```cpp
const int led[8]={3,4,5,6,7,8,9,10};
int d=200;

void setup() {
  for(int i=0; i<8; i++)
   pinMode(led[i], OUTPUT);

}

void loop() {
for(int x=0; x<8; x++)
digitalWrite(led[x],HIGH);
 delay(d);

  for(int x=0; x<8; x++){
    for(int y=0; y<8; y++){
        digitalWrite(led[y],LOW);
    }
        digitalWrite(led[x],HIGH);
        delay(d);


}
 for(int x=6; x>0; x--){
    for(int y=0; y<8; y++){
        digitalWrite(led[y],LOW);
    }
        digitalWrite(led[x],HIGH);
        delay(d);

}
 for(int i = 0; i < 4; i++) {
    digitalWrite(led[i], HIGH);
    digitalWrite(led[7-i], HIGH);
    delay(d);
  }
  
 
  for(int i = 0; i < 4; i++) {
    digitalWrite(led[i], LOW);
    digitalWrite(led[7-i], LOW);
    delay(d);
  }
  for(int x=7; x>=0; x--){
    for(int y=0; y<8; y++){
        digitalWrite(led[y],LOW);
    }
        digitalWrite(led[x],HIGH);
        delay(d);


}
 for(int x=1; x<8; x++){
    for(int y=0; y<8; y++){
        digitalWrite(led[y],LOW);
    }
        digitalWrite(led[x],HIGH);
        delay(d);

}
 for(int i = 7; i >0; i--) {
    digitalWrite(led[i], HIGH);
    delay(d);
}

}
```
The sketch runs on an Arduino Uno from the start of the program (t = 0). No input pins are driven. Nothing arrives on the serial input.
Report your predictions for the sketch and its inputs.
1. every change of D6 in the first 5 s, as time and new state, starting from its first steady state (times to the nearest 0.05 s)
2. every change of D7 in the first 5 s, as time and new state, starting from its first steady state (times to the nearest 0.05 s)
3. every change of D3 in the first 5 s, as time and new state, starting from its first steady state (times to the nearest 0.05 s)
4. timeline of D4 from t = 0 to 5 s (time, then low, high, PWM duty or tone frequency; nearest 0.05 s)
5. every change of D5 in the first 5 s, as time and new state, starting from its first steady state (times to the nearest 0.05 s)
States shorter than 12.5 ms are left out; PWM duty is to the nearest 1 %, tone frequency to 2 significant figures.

0 s high; 0.2 s low; 0.8 s high; 1 s low; 2.4 s high; 2.6 s low; 3.6 s high; 4.4 s low
0 s high; 0.2 s low; 1 s high; 1.2 s low; 2.2 s high; 2.4 s low; 3.6 s high; 4.4 s low
0 s high; 0.4 s low; 3 s high; 3.8 s low
0 s high; 0.2 s low; 0.4 s high; 0.6 s low; 2.8 s high; 4 s low
0 s high; 0.2 s low; 0.6 s high; 0.8 s low; 2.6 s high; 2.8 s low; 3.4 s high; 4.2 s low
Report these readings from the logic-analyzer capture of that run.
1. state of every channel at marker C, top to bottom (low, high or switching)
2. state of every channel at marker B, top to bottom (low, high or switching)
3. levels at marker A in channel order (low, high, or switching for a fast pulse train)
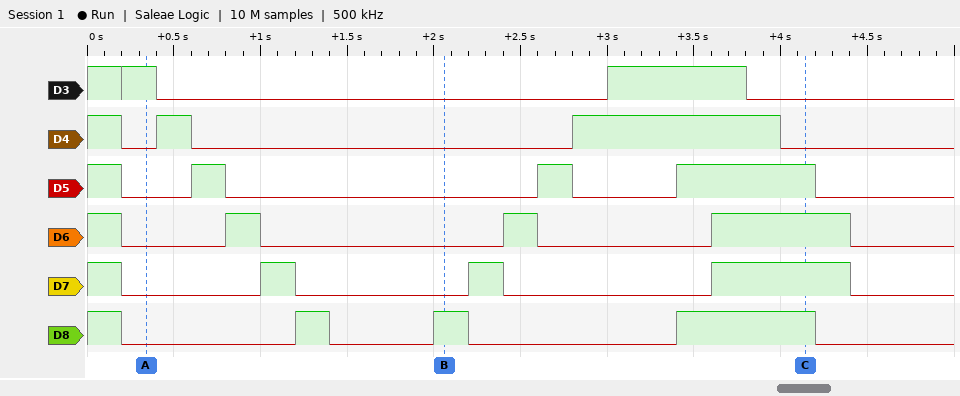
D3 low, D4 low, D5 high, D6 high, D7 high, D8 high
D3 low, D4 low, D5 low, D6 low, D7 low, D8 high
D3 high, D4 low, D5 low, D6 low, D7 low, D8 low
